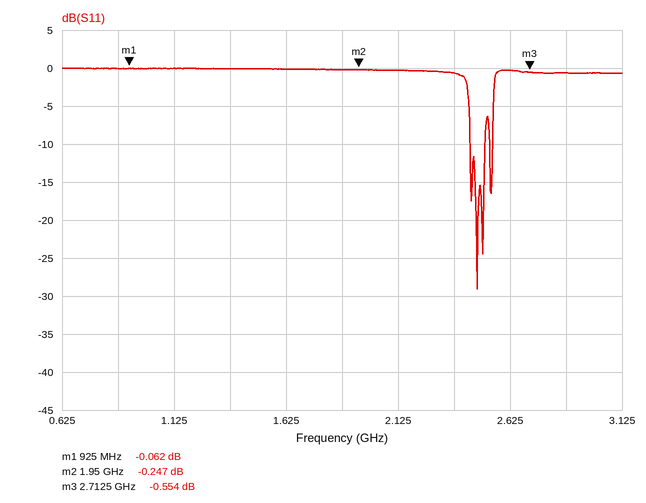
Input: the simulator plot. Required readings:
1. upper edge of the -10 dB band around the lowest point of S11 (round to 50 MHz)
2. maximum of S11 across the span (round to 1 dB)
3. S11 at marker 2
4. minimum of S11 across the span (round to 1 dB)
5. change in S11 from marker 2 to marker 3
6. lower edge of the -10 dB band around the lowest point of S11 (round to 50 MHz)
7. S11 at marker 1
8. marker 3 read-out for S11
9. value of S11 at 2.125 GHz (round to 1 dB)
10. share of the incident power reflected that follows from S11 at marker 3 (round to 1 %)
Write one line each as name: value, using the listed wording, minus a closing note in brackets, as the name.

upper edge of the -10 dB band around the lowest point of S11: 2.50 GHz
maximum of S11 across the span: 0 dB
S11 at marker 2: -0.247 dB
minimum of S11 across the span: -29 dB
change in S11 from marker 2 to marker 3: -0.307 dB
lower edge of the -10 dB band around the lowest point of S11: 2.45 GHz
S11 at marker 1: -0.062 dB
marker 3 read-out for S11: -0.554 dB
value of S11 at 2.125 GHz: 0 dB
share of the incident power reflected that follows from S11 at marker 3: 88 %
